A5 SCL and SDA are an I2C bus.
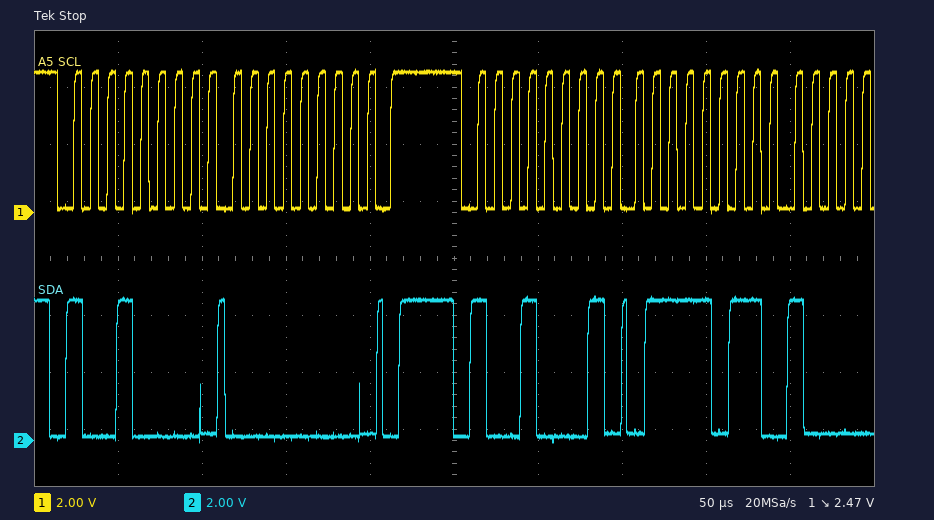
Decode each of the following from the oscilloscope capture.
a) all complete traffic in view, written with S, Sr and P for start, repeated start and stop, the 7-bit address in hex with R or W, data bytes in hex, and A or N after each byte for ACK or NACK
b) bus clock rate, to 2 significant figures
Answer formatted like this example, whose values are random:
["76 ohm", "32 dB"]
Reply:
["S 48W A 00 A P S 48R A 7B A", "100 kHz"]
